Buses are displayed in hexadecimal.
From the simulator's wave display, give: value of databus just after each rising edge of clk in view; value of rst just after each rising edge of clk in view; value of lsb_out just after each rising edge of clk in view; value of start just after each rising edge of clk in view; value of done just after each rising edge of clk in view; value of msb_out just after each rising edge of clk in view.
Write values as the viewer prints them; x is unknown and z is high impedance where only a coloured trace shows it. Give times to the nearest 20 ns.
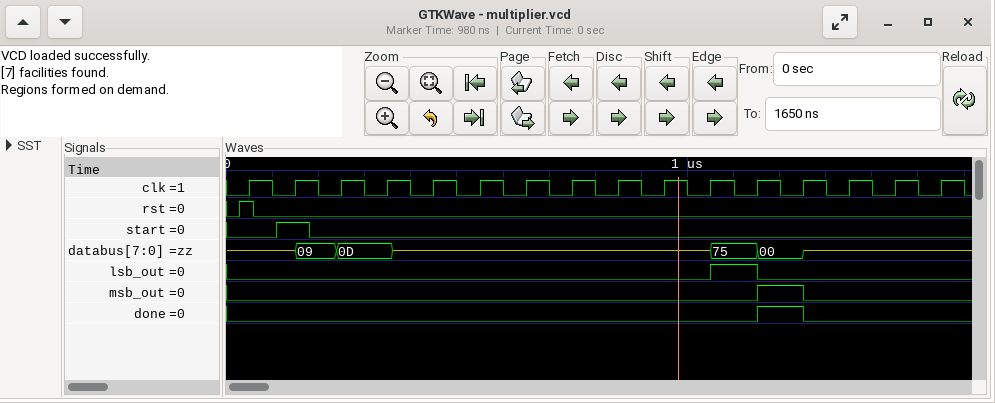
z, 09, 0D, 0D, z, z, z, z, z, z, 75, 00, z, z, z, z
1 0 0 0 0 0 0 0 0 0 0 0 0 0 0 0
0 0 0 0 0 0 0 0 0 0 1 0 0 0 0 0
0 1 0 0 0 0 0 0 0 0 0 0 0 0 0 0
0 0 0 0 0 0 0 0 0 0 0 1 0 0 0 0
0 0 0 0 0 0 0 0 0 0 0 1 0 0 0 0
